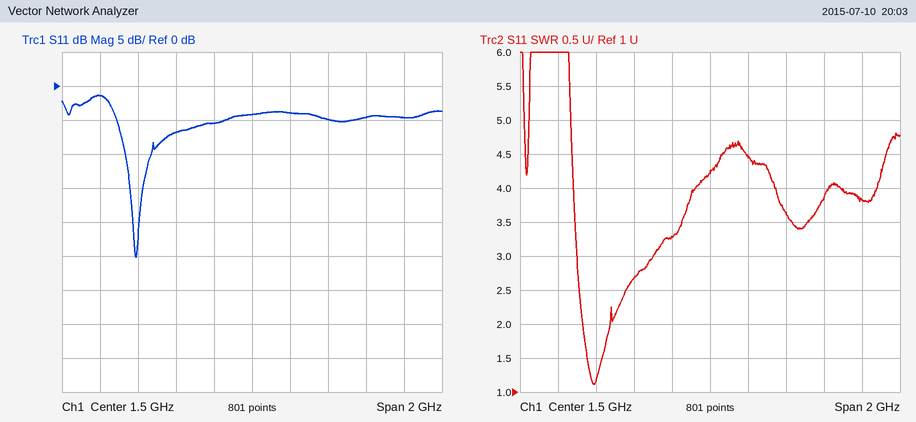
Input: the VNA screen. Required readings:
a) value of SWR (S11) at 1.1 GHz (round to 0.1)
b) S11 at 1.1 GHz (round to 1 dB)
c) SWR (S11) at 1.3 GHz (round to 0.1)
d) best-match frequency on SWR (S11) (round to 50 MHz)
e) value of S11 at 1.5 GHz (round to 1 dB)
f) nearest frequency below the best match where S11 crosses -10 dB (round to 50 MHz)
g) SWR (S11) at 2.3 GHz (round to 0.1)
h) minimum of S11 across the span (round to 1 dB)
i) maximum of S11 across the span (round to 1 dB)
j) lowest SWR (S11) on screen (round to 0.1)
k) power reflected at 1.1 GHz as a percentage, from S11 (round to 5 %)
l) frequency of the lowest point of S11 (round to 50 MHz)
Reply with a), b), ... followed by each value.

a) 2.7
b) -7 dB
c) 3.3
d) 900 MHz
e) -4 dB
f) 850 MHz
g) 3.8
h) -25 dB
i) -1 dB
j) 1.1
k) 20 %
l) 900 MHz
